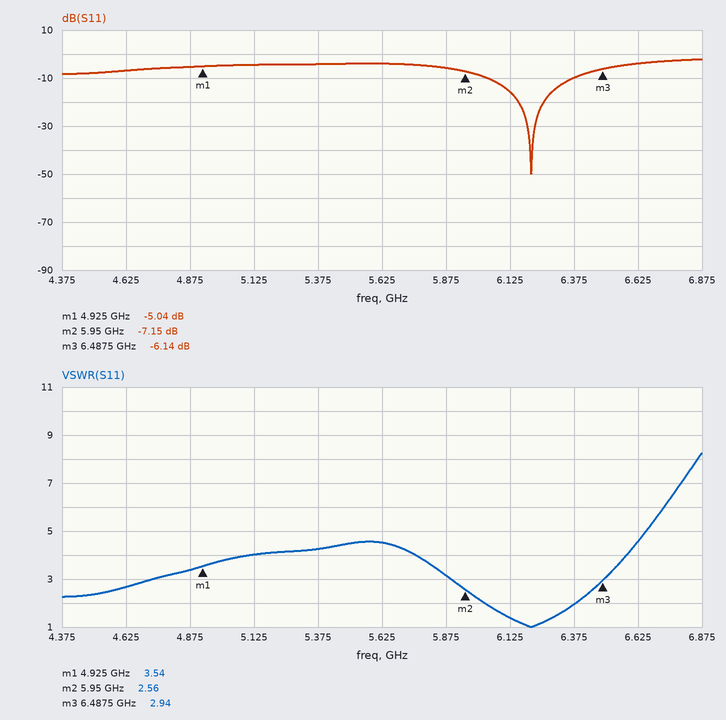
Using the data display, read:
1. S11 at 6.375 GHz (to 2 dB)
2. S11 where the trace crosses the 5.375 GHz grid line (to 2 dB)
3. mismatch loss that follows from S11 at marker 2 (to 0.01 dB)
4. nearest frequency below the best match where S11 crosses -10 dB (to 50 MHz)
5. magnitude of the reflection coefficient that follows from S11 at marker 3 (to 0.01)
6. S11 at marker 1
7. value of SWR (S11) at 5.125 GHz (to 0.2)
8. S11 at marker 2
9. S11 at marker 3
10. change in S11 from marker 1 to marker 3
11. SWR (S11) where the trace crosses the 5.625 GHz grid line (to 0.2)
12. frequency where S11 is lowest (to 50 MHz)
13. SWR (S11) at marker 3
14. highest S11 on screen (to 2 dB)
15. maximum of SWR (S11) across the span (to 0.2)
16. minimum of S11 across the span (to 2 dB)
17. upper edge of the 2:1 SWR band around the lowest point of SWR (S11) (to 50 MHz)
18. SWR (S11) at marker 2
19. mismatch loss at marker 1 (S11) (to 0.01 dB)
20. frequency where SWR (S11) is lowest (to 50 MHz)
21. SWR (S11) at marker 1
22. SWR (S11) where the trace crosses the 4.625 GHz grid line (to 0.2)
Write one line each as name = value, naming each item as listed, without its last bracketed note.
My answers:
S11 at 6.375 GHz = -10 dB
S11 where the trace crosses the 5.375 GHz grid line = -4 dB
mismatch loss that follows from S11 at marker 2 = 0.93 dB
nearest frequency below the best match where S11 crosses -10 dB = 6.05 GHz
magnitude of the reflection coefficient that follows from S11 at marker 3 = 0.49
S11 at marker 1 = -5.04 dB
value of SWR (S11) at 5.125 GHz = 4.0
S11 at marker 2 = -7.15 dB
S11 at marker 3 = -6.14 dB
change in S11 from marker 1 to marker 3 = -1.10 dB
SWR (S11) where the trace crosses the 5.625 GHz grid line = 4.6
frequency where S11 is lowest = 6.20 GHz
SWR (S11) at marker 3 = 2.94
highest S11 on screen = -2 dB
maximum of SWR (S11) across the span = 8.2
minimum of S11 across the span = -50 dB
upper edge of the 2:1 SWR band around the lowest point of SWR (S11) = 6.40 GHz
SWR (S11) at marker 2 = 2.56
mismatch loss at marker 1 (S11) = 1.63 dB
frequency where SWR (S11) is lowest = 6.20 GHz
SWR (S11) at marker 1 = 3.54
SWR (S11) where the trace crosses the 4.625 GHz grid line = 2.6
